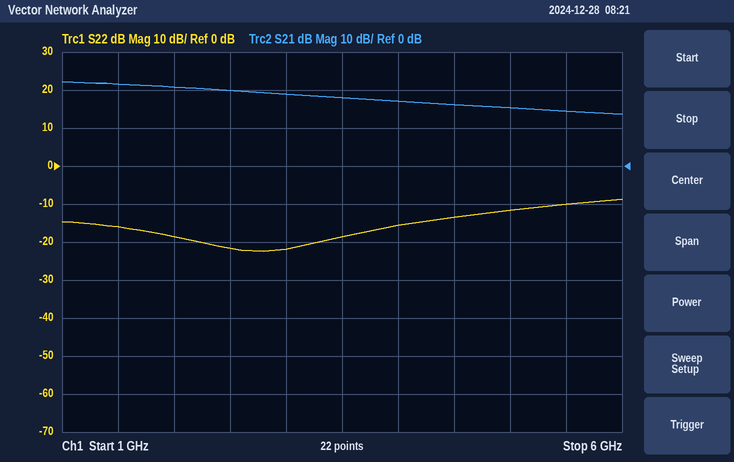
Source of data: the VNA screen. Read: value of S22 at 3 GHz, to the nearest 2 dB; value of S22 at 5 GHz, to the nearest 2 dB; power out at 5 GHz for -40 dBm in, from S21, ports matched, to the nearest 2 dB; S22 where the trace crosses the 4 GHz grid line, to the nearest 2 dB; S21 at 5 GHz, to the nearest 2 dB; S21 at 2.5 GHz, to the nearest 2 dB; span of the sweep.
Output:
-22 dB
-12 dB
-24 dBm
-16 dB
16 dB
20 dB
5 GHz
